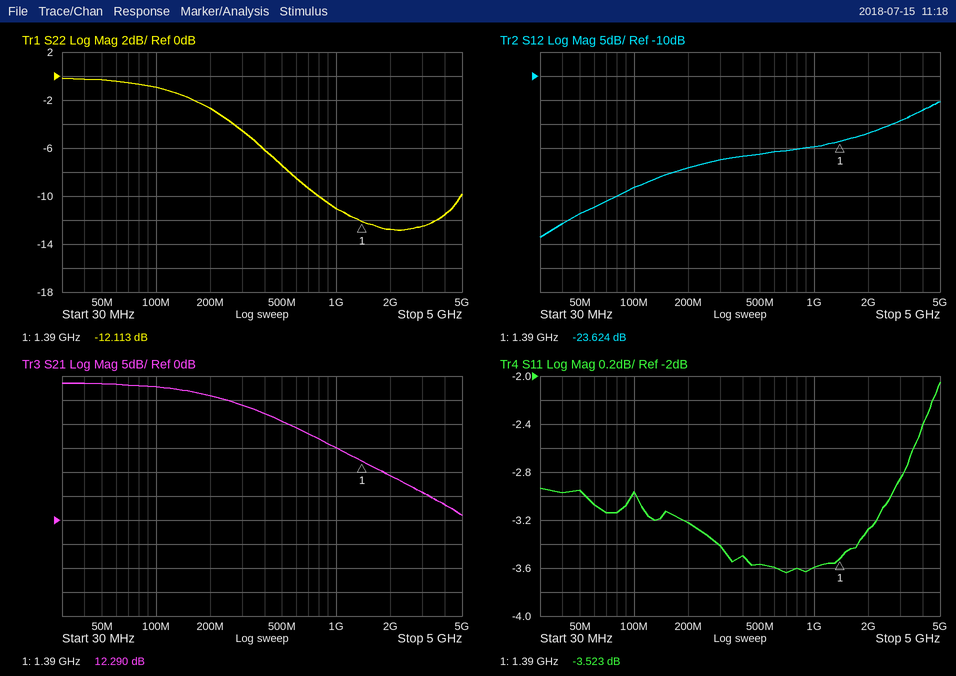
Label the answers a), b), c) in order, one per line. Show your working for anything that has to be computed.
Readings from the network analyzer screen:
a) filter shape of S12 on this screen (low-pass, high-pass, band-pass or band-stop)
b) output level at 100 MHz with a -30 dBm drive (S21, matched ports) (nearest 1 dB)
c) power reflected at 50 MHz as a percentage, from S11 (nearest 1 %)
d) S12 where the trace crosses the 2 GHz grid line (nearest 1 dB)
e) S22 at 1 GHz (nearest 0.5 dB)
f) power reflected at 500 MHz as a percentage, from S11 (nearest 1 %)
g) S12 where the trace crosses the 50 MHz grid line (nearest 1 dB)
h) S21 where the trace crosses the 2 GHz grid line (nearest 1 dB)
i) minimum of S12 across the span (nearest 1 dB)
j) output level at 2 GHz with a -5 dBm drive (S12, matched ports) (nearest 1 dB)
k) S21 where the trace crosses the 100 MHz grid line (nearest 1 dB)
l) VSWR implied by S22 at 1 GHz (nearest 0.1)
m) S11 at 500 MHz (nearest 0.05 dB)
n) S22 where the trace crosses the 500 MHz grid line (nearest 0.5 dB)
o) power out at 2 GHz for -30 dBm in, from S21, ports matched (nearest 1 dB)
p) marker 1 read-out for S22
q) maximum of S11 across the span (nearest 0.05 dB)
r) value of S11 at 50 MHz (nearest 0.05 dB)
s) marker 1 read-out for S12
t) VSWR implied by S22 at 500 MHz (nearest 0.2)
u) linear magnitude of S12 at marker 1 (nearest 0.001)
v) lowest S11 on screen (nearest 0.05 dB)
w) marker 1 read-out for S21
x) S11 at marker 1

a) high-pass
b) -30 dBm + (28 dB) = -2 dBm
c) 10^(-2.95/10) ≈ 51 %
d) -22 dB
e) -11.0 dB
f) 10^(-3.55/10) ≈ 44 %
g) -39 dB
h) 9 dB
i) -44 dB
j) -5 dBm + (-22 dB) = -27 dBm
k) 28 dB
l) |Γ| = 10^(-11/20) = 0.2818; VSWR = (1 + 0.2818)/(1 − 0.2818) ≈ 1.8
m) -3.55 dB
n) -7.5 dB
o) -30 dBm + (9 dB) = -21 dBm
p) -12.113 dB
q) -2.05 dB
r) -2.95 dB
s) -23.624 dB
t) |Γ| = 10^(-7.5/20) = 0.4217; VSWR = (1 + 0.4217)/(1 − 0.4217) ≈ 2.46, so 2.4 to the nearest 0.2
u) 10^(-23.624/20) ≈ 0.066
v) -3.65 dB
w) 12.290 dB
x) -3.523 dB
